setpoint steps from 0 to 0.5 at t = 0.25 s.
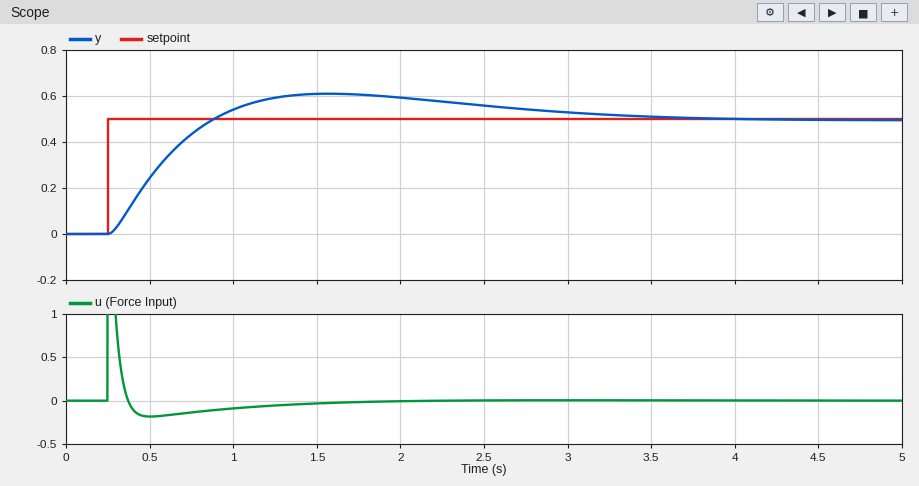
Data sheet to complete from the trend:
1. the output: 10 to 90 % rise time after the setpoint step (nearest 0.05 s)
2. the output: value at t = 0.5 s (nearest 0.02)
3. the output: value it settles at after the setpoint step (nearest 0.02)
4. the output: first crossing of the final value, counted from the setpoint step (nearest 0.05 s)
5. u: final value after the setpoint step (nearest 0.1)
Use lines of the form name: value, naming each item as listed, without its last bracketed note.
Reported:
the output: 10 to 90 % rise time after the setpoint step: 0.45 s
the output: value at t = 0.5 s: 0.24
the output: value it settles at after the setpoint step: 0.50
the output: first crossing of the final value, counted from the setpoint step: 0.65 s
u: final value after the setpoint step: 0.0
